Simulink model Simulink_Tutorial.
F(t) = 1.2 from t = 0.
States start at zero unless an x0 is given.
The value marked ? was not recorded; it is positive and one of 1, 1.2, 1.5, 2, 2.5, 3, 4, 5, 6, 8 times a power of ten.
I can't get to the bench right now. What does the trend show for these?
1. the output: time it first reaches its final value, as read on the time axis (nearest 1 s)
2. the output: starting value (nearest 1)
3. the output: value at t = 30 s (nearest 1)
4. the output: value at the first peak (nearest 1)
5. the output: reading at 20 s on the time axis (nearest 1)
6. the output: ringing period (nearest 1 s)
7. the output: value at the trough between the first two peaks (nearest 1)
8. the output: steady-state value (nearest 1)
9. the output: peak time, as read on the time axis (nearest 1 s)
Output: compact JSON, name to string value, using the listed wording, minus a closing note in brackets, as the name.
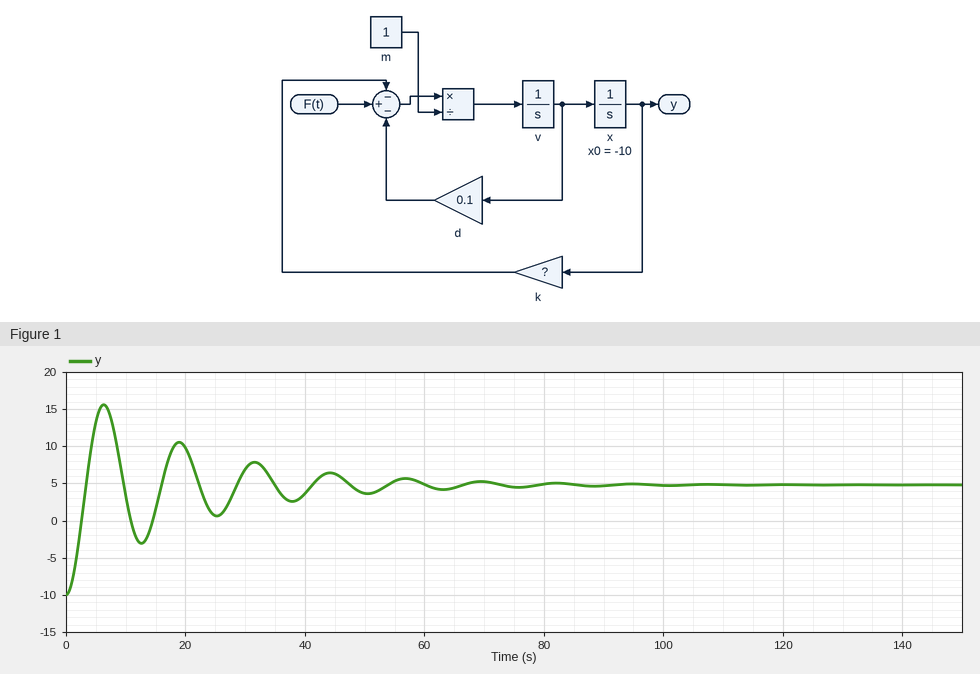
{"the output: time it first reaches its final value, as read on the time axis": "3 s", "the output: starting value": "-10", "the output: value at t = 30 s": "7", "the output: value at the first peak": "16", "the output: reading at 20 s on the time axis": "10", "the output: ringing period": "13 s", "the output: value at the trough between the first two peaks": "-3", "the output: steady-state value": "5", "the output: peak time, as read on the time axis": "6 s"}
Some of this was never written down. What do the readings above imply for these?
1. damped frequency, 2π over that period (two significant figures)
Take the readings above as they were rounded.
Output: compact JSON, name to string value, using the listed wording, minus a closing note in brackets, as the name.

{"damped frequency, 2π over that period": "0.48 rad/s"}
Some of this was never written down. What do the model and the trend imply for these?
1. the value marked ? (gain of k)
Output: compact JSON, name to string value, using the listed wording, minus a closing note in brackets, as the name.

{"the value marked ?": "0.25"}
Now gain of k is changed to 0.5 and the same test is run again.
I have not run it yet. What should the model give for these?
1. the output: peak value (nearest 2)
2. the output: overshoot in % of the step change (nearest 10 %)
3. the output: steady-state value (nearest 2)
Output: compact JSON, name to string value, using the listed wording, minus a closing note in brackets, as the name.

{"the output: peak value": "12", "the output: overshoot in % of the step change": "80 %", "the output: steady-state value": "2"}
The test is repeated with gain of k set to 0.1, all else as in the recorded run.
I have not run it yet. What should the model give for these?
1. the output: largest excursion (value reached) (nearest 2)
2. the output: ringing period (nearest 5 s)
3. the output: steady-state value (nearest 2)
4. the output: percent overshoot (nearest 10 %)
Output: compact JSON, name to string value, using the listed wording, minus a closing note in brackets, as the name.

{"the output: largest excursion (value reached)": "26", "the output: ringing period": "20 s", "the output: steady-state value": "12", "the output: percent overshoot": "60 %"}
